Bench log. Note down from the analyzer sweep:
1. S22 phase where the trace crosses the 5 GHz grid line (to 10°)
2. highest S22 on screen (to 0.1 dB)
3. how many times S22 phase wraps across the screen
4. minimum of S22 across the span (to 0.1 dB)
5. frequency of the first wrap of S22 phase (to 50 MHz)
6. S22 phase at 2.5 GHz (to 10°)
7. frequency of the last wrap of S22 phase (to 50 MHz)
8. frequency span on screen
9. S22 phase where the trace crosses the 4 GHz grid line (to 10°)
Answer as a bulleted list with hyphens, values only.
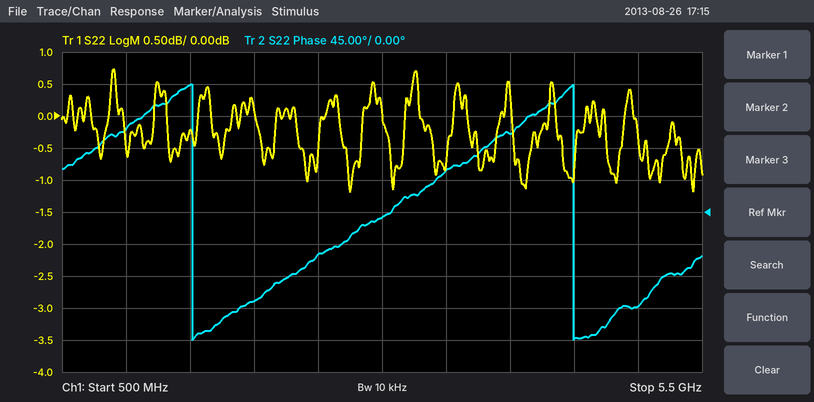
- -130°
- 0.7 dB
- 2
- -1.2 dB
- 1.50 GHz
- -60°
- 4.50 GHz
- 5 GHz
- 110°
